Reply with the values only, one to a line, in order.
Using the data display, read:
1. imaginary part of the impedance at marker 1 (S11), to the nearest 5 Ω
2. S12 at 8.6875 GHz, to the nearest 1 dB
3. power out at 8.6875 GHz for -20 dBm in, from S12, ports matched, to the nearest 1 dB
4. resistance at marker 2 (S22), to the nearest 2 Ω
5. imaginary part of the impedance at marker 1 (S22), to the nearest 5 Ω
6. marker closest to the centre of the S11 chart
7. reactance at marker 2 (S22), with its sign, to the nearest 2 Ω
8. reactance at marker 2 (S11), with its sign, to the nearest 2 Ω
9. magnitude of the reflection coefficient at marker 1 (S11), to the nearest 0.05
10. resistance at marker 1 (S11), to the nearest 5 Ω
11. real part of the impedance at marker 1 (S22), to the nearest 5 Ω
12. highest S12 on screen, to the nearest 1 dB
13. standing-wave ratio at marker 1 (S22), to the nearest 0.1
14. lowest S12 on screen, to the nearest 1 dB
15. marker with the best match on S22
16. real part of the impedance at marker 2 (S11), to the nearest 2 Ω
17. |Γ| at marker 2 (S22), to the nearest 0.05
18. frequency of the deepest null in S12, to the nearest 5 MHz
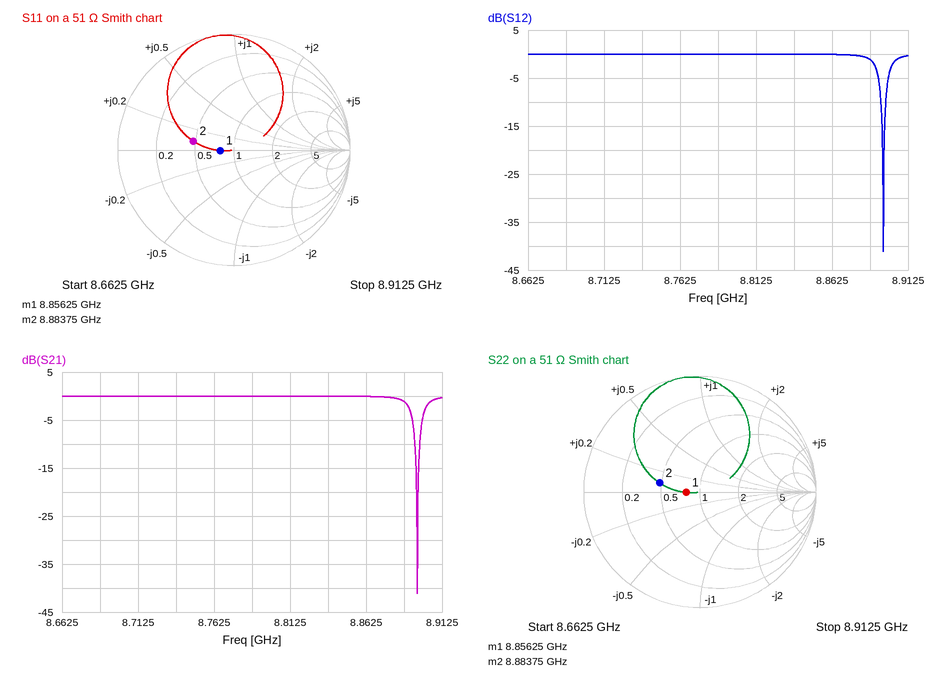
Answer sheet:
0 Ω
0 dB
-20 dBm
24 Ω
0 Ω
marker 1
+4 Ω
+4 Ω
0.10
40 Ω
40 Ω
0 dB
1.3
-41 dB
marker 1
24 Ω
0.35
8.895 GHz
